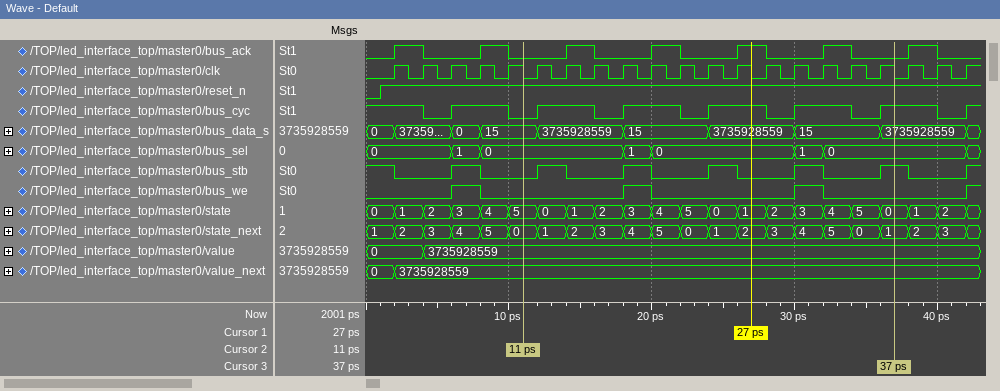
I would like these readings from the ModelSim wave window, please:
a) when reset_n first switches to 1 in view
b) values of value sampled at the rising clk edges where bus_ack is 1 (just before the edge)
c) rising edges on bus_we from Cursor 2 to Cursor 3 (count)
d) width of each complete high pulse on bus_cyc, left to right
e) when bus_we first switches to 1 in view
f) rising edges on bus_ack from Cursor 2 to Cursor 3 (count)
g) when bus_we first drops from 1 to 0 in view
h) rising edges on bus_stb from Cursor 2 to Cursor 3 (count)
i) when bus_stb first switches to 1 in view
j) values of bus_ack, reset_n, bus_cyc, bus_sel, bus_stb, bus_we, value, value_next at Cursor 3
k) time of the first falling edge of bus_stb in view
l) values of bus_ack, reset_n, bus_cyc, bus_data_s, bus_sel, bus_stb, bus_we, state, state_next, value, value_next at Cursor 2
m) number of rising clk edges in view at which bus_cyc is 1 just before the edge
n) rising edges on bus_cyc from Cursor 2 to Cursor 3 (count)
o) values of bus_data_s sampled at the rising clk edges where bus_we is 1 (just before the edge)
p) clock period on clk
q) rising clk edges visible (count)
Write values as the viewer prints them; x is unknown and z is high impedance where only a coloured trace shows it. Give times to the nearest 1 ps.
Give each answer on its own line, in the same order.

1 ps
0, 3735928559, 3735928559, 3735928559, 3735928559, 3735928559, 3735928559
2
4 ps, 4 ps, 4 ps, 4 ps, 4 ps, 4 ps
6 ps
4
8 ps
5
6 ps
bus_ack=0, reset_n=1, bus_cyc=1, bus_sel=0, bus_stb=1, bus_we=0, value=3735928559, value_next=3735928559
2 ps
bus_ack=0, reset_n=1, bus_cyc=0, bus_data_s=15, bus_sel=0, bus_stb=0, bus_we=0, state=5, state_next=0, value=3735928559, value_next=3735928559
14
5
0, 15, 15
2 ps
21
